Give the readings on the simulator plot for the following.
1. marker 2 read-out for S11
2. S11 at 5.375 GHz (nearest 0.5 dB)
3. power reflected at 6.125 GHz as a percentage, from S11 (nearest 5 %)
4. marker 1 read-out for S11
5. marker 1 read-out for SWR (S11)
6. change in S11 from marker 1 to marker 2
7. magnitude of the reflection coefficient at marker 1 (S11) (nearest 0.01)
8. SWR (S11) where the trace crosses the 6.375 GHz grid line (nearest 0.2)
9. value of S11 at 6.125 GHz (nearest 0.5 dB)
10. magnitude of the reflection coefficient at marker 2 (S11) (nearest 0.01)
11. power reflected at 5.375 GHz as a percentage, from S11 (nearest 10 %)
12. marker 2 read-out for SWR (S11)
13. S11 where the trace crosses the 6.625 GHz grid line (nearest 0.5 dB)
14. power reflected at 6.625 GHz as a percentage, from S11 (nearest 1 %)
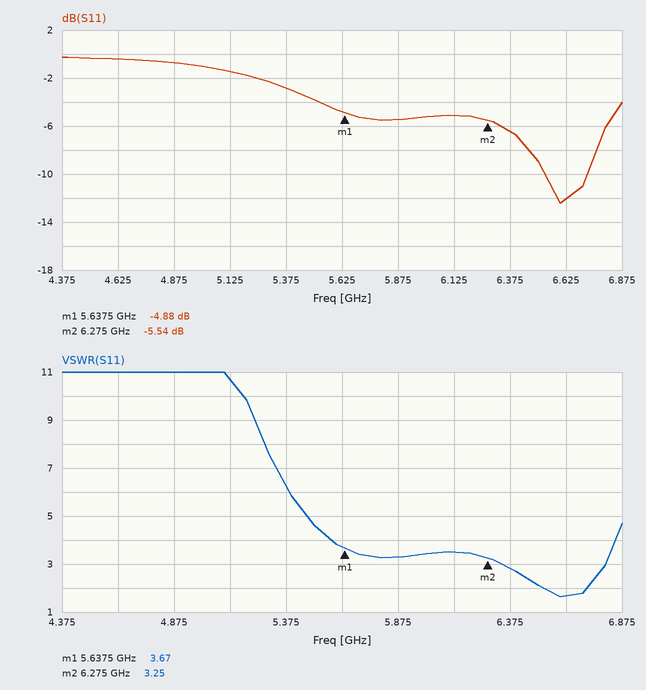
-5.54 dB
-3.0 dB
30 %
-4.88 dB
3.67
-0.66 dB
0.57
2.8
-5.0 dB
0.53
50 %
3.25
-12.0 dB
6 %
